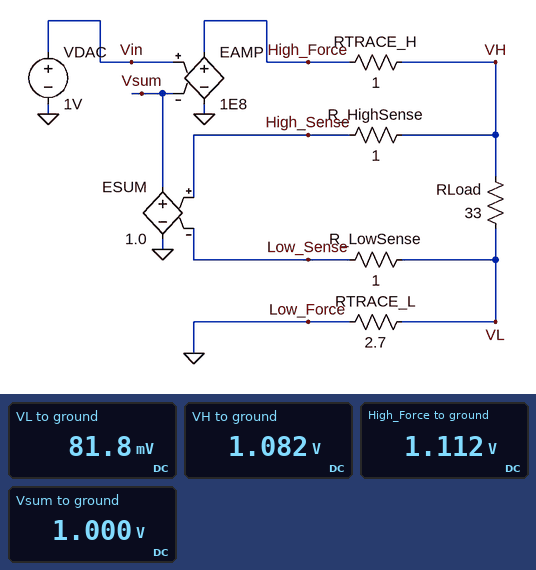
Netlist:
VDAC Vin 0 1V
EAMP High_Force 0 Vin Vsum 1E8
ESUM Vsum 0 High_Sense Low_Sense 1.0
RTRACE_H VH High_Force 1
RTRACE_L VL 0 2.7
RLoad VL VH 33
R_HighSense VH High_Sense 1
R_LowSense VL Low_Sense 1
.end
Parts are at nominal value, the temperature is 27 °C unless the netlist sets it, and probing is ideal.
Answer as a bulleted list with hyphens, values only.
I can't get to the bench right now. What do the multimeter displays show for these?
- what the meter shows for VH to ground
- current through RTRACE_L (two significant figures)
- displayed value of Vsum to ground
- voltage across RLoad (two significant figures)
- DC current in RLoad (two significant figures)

- 1.082 V
- 30 mA
- 1.000 V
- 1.0 V
- 30 mA
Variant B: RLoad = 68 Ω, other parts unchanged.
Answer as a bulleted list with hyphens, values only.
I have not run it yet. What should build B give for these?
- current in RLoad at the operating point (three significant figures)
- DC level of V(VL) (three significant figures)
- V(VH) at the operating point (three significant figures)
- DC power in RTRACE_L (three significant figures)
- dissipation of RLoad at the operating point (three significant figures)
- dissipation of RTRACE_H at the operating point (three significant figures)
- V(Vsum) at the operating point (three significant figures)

- 14.7 mA
- 39.7 mV
- 1.04 V
- 584 µW
- 14.7 mW
- 216 µW
- 1.00 V
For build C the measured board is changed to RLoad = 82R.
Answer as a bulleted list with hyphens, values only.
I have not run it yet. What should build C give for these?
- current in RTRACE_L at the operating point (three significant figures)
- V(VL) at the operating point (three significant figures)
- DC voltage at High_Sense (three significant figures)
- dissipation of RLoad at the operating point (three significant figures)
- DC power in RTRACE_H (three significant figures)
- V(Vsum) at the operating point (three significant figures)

- 12.2 mA
- 32.9 mV
- 1.03 V
- 12.2 mW
- 149 µW
- 1.00 V
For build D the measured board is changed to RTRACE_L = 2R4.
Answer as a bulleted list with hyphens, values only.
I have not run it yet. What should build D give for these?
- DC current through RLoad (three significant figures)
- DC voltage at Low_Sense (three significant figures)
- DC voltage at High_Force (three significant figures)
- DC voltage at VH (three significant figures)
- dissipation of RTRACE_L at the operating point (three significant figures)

- 30.3 mA
- 72.7 mV
- 1.10 V
- 1.07 V
- 2.20 mW
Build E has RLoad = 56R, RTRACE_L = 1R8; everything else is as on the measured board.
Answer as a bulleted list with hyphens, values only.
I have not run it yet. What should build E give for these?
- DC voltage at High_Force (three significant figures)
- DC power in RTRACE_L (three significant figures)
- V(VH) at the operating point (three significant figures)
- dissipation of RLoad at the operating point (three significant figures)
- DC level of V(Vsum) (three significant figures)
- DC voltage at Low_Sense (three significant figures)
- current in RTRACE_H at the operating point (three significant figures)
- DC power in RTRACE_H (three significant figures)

- 1.05 V
- 574 µW
- 1.03 V
- 17.9 mW
- 1.00 V
- 32.1 mV
- 17.9 mA
- 319 µW
